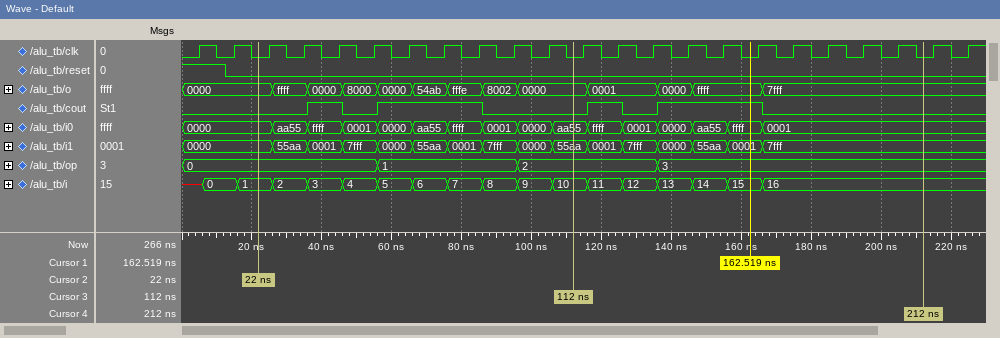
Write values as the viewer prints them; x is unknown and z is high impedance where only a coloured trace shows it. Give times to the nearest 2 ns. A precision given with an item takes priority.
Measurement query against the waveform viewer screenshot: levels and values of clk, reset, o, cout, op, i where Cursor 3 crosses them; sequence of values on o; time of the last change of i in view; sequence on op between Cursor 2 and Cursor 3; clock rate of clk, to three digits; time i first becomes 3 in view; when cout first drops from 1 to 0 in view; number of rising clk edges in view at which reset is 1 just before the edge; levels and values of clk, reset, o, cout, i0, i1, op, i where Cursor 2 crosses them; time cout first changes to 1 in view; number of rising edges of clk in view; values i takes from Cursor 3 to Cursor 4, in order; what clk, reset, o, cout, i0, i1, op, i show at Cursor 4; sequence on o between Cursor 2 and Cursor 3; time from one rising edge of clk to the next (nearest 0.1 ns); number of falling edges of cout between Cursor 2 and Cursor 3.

clk=0, reset=0, o=0000, cout=0, op=2, i=10
0000, ffff, 0000, 8000, 0000, 54ab, fffe, 8002, 0000, 0001, 0000, ffff, 7fff
166 ns
0, 1, 2
100 MHz
36 ns
46 ns
1
clk=0, reset=0, o=0000, cout=0, i0=0000, i1=0000, op=0, i=1
36 ns
23
10, 11, 12, 13, 14, 15, 16
clk=0, reset=0, o=7fff, cout=0, i0=0001, i1=7fff, op=3, i=16
0000, ffff, 0000, 8000, 0000, 54ab, fffe, 8002, 0000
10 ns
2
